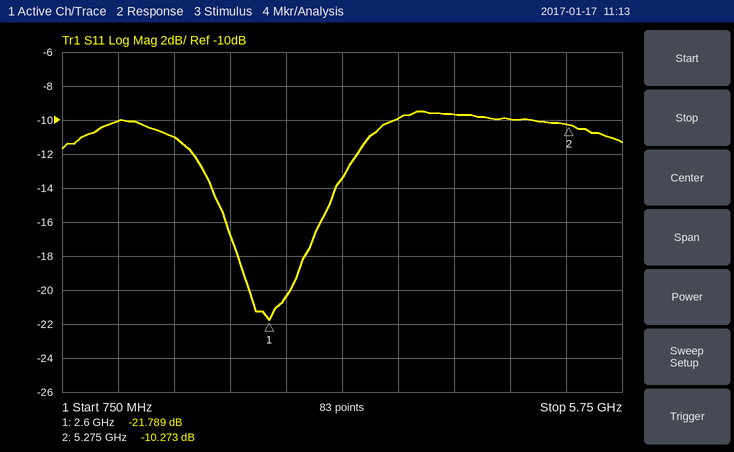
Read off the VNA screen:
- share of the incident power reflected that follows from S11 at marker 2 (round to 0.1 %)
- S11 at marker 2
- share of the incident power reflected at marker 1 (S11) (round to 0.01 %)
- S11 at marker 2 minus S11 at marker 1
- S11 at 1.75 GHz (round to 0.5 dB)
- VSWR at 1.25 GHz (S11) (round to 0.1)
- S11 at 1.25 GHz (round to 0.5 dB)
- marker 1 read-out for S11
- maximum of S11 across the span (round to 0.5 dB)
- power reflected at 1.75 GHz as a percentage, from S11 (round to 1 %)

9.4 %
-10.273 dB
0.66 %
11.516 dB
-11.0 dB
1.9
-10.0 dB
-21.789 dB
-9.5 dB
8 %
